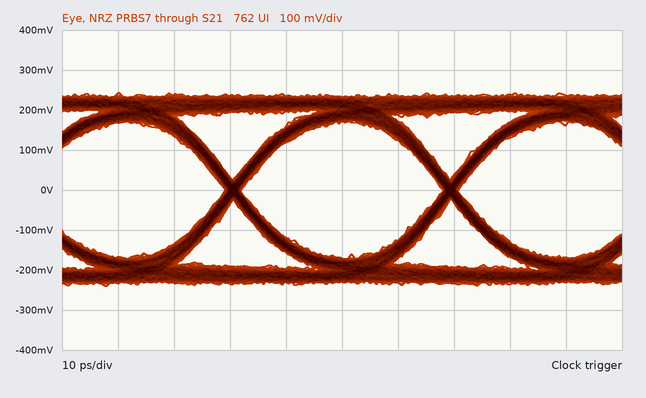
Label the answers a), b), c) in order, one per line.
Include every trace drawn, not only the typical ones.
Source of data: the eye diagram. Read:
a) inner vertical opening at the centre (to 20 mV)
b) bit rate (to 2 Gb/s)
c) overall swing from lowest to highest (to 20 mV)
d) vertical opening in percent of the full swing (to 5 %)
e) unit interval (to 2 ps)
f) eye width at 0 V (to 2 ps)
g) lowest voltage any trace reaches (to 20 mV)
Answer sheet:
a) 340 mV
b) 26 Gb/s
c) 480 mV
d) 70 %
e) 38 ps
f) 36 ps
g) -240 mV
